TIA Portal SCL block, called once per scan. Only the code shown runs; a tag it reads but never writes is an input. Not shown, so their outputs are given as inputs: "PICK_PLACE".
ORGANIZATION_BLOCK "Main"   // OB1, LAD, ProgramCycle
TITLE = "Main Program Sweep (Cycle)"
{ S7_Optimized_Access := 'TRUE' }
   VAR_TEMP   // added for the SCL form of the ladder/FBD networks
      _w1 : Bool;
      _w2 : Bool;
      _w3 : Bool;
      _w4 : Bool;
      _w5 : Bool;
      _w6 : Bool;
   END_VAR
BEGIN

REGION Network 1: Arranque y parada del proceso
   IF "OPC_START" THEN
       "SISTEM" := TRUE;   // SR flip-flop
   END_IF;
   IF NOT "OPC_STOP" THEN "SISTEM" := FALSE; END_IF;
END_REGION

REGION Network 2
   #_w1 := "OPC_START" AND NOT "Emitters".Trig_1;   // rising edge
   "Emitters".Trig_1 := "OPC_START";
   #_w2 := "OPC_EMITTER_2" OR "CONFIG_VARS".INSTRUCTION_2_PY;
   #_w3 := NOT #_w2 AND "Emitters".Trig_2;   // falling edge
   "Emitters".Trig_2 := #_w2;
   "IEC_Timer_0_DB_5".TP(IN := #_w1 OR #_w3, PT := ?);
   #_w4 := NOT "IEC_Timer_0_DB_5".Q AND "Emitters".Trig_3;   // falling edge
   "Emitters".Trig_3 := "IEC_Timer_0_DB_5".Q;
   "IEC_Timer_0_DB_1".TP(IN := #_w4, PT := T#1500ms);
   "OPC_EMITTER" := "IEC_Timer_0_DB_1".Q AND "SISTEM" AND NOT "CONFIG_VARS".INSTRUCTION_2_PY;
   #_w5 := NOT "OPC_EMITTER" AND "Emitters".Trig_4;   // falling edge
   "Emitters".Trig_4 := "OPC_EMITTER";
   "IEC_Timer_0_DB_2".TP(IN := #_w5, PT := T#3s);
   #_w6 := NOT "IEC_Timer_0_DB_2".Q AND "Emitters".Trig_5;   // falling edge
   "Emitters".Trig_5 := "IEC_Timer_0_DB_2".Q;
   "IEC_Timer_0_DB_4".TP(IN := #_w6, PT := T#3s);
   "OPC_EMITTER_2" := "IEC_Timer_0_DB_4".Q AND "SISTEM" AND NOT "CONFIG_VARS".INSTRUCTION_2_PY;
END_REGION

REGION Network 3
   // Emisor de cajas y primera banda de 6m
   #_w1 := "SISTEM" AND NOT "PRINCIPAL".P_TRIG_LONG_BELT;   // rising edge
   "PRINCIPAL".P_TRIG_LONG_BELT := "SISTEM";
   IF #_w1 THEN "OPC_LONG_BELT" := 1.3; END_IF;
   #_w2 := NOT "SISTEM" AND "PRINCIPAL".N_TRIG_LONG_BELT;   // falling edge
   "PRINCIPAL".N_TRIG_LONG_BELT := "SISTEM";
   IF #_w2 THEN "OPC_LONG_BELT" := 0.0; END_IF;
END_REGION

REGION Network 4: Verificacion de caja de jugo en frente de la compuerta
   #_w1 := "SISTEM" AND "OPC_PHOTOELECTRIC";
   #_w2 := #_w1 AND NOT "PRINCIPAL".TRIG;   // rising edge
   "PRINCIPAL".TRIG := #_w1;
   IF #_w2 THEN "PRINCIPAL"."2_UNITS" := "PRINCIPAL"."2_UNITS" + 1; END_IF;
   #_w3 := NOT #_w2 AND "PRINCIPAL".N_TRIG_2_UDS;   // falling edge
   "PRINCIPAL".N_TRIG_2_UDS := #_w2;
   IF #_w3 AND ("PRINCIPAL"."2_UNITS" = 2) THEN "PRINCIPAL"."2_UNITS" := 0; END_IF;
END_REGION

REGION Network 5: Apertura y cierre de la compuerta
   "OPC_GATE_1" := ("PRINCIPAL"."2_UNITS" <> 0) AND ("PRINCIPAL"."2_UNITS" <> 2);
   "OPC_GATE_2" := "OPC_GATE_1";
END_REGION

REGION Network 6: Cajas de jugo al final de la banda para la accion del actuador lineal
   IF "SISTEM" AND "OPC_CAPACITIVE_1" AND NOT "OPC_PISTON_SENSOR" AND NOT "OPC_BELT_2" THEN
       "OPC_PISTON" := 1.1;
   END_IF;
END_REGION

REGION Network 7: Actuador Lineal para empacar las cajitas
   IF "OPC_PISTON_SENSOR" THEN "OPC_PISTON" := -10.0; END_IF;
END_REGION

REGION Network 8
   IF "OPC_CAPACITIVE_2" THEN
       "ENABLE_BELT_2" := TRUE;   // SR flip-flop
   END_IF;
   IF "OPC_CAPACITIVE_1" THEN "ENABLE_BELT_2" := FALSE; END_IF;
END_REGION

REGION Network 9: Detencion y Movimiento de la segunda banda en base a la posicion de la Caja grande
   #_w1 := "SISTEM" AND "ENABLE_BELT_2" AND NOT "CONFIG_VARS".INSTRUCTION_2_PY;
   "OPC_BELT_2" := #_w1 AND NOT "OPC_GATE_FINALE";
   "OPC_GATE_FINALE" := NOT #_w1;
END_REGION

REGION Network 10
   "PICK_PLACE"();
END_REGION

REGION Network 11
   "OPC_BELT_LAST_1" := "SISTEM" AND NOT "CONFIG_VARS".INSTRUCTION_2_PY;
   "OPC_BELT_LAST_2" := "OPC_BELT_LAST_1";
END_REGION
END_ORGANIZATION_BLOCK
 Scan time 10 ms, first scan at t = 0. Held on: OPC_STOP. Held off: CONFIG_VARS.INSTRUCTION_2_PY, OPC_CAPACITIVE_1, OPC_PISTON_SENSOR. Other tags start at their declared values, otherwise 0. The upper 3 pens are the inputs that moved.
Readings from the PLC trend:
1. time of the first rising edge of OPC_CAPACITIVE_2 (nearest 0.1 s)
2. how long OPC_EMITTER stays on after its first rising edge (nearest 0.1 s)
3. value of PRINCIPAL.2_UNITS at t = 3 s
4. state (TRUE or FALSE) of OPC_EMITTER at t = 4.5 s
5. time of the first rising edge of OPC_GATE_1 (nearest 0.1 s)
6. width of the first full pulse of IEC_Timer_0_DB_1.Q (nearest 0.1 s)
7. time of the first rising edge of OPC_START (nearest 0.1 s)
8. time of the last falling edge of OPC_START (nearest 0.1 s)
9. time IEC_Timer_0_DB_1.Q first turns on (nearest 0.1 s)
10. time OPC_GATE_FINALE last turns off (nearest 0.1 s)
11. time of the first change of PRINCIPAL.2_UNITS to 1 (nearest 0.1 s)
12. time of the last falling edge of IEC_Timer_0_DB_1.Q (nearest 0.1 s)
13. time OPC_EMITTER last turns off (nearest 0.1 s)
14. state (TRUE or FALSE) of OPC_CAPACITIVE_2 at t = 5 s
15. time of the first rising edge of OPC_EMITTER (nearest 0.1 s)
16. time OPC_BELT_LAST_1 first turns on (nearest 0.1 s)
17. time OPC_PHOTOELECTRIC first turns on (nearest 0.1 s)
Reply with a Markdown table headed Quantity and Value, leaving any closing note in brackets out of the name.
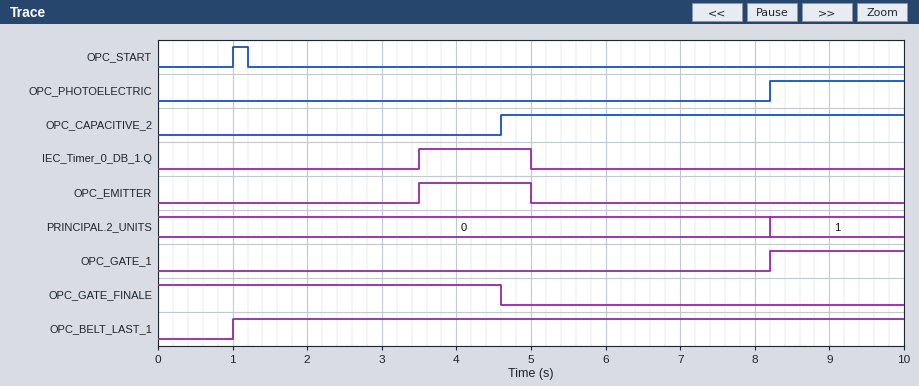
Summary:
| Quantity | Value |
|---|---|
| time of the first rising edge of OPC_CAPACITIVE_2 | 4.6 s |
| how long OPC_EMITTER stays on after its first rising edge | 1.5 s |
| value of PRINCIPAL.2_UNITS at t = 3 s | 0 |
| state (TRUE or FALSE) of OPC_EMITTER at t = 4.5 s | TRUE |
| time of the first rising edge of OPC_GATE_1 | 8.2 s |
| width of the first full pulse of IEC_Timer_0_DB_1.Q | 1.5 s |
| time of the first rising edge of OPC_START | 1.0 s |
| time of the last falling edge of OPC_START | 1.2 s |
| time IEC_Timer_0_DB_1.Q first turns on | 3.5 s |
| time OPC_GATE_FINALE last turns off | 4.6 s |
| time of the first change of PRINCIPAL.2_UNITS to 1 | 8.2 s |
| time of the last falling edge of IEC_Timer_0_DB_1.Q | 5.0 s |
| time OPC_EMITTER last turns off | 5.0 s |
| state (TRUE or FALSE) of OPC_CAPACITIVE_2 at t = 5 s | TRUE |
| time of the first rising edge of OPC_EMITTER | 3.5 s |
| time OPC_BELT_LAST_1 first turns on | 1.0 s |
| time OPC_PHOTOELECTRIC first turns on | 8.2 s |
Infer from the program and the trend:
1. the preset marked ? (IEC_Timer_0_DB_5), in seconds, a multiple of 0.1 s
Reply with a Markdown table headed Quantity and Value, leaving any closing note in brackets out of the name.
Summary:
| Quantity | Value |
|---|---|
| the preset marked ? (IEC_Timer_0_DB_5), in seconds, a multiple of 0.1 s | 2.5 s |
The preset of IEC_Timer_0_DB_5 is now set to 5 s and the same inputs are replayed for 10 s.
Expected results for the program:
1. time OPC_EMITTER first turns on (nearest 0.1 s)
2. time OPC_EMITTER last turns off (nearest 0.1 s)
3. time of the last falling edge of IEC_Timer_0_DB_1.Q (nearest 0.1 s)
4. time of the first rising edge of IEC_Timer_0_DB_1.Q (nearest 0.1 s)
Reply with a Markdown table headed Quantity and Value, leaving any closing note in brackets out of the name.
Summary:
| Quantity | Value |
|---|---|
| time OPC_EMITTER first turns on | 6.0 s |
| time OPC_EMITTER last turns off | 7.5 s |
| time of the last falling edge of IEC_Timer_0_DB_1.Q | 7.5 s |
| time of the first rising edge of IEC_Timer_0_DB_1.Q | 6.0 s |
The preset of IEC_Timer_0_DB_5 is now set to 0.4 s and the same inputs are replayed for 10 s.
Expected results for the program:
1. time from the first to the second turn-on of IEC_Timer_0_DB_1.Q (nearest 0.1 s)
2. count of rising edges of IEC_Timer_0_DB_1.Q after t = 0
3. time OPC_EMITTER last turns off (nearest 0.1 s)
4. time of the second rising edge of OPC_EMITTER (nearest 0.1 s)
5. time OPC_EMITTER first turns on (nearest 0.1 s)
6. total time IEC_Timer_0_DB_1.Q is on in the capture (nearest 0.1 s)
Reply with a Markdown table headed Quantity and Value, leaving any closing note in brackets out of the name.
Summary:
| Quantity | Value |
|---|---|
| time from the first to the second turn-on of IEC_Timer_0_DB_1.Q | 7.9 s |
| count of rising edges of IEC_Timer_0_DB_1.Q after t = 0 | 2 |
| time OPC_EMITTER last turns off | 2.9 s |
| time of the second rising edge of OPC_EMITTER | 9.3 s |
| time OPC_EMITTER first turns on | 1.4 s |
| total time IEC_Timer_0_DB_1.Q is on in the capture | 2.2 s |
